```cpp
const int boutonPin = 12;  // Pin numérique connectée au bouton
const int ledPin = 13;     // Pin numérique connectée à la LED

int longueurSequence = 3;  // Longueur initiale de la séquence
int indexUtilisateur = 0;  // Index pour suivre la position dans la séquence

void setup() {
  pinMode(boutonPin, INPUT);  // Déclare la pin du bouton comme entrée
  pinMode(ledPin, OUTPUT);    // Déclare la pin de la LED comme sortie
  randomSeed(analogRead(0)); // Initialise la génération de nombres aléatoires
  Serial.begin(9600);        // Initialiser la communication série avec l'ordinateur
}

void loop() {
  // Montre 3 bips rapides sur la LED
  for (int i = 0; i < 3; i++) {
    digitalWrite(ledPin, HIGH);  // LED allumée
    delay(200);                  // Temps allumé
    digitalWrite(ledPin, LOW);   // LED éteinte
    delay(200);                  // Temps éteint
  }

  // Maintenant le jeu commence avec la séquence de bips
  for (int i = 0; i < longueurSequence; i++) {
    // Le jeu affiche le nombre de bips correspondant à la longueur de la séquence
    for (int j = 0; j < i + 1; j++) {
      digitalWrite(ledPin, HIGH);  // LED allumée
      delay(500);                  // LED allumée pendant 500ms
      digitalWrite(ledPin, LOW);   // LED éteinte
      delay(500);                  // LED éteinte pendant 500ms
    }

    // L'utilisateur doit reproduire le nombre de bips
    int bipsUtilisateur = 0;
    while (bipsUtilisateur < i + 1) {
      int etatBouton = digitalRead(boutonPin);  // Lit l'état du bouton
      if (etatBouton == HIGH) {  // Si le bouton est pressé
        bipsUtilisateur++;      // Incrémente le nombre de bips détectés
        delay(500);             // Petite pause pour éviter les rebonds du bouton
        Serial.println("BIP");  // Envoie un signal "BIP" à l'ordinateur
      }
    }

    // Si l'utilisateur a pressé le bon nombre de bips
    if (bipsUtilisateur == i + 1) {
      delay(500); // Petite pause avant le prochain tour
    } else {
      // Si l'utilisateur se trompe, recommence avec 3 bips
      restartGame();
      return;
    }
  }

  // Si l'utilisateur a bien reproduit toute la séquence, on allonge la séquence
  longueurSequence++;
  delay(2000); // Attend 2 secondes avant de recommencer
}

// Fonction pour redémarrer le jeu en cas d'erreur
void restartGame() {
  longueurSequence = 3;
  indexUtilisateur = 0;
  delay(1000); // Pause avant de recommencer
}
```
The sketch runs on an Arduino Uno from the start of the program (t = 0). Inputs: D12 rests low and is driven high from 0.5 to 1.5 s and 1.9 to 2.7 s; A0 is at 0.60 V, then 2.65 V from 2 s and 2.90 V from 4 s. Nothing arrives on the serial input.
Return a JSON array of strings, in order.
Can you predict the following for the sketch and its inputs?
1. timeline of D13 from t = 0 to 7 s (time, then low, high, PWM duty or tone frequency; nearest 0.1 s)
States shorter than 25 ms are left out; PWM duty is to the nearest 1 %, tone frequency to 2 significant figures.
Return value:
["0 s high; 0.2 s low; 0.4 s high; 0.6 s low; 0.8 s high; 1 s low; 1.2 s high; 1.7 s low; 3.2 s high; 3.7 s low; 4.2 s high; 4.7 s low"]
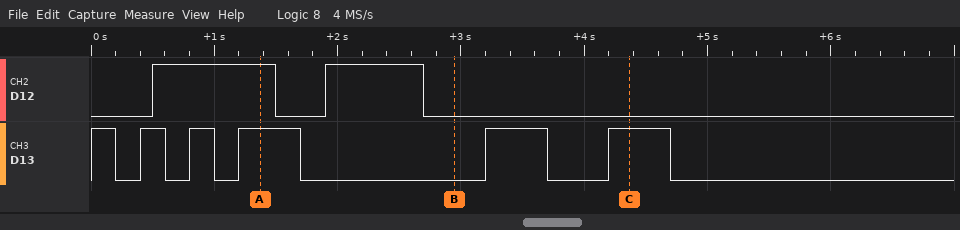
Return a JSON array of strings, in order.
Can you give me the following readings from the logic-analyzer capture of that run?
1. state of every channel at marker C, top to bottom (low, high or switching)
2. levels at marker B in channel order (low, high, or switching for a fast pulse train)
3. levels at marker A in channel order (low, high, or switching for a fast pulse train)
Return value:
["D12 low, D13 high", "D12 low, D13 low", "D12 high, D13 high"]
